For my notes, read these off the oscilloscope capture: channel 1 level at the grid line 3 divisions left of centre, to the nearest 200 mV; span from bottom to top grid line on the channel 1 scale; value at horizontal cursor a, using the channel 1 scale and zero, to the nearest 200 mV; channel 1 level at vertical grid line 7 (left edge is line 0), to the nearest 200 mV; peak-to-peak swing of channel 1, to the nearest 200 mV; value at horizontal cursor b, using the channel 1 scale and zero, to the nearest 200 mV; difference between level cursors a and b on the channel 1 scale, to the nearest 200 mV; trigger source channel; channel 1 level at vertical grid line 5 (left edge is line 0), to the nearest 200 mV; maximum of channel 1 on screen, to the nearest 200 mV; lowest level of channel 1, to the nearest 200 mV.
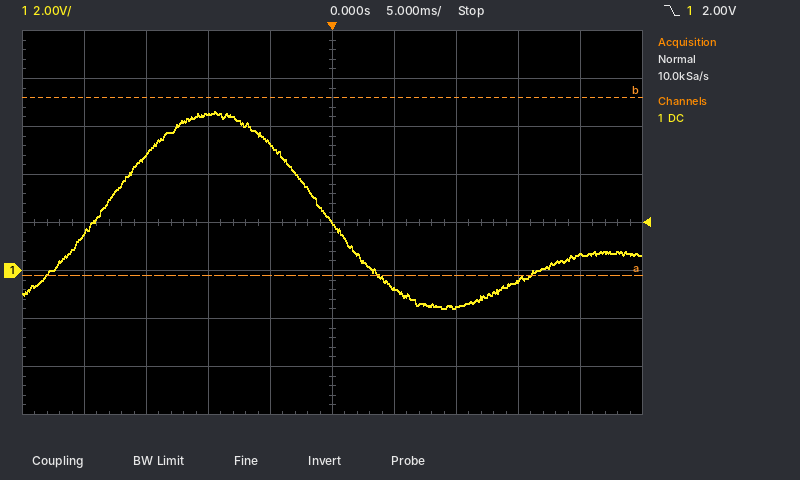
4.8 V
16 V
-200 mV
-1.6 V
8.2 V
7.2 V
7.4 V
channel 1
2.0 V
6.6 V
-1.6 V
